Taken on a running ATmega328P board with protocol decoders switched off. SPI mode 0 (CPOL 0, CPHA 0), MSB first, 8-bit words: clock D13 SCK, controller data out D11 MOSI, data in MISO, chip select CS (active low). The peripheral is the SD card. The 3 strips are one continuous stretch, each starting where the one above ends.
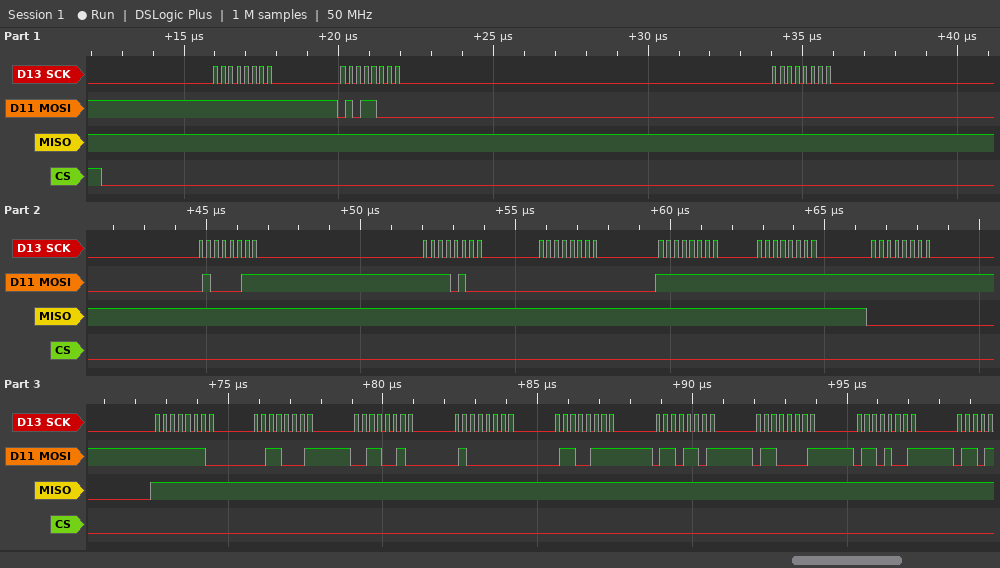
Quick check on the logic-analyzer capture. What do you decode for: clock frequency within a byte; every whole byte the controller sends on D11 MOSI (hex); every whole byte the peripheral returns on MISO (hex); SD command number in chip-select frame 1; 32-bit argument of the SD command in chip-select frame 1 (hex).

4 MHz
FF 58 00 43 F4 00 FF FF FF FE 31 32 40 67 6D 61 69
FF FF FF FF FF FF FF FF 00 FF FF FF FF FF FF FF FF
CMD24
0x0043F400
